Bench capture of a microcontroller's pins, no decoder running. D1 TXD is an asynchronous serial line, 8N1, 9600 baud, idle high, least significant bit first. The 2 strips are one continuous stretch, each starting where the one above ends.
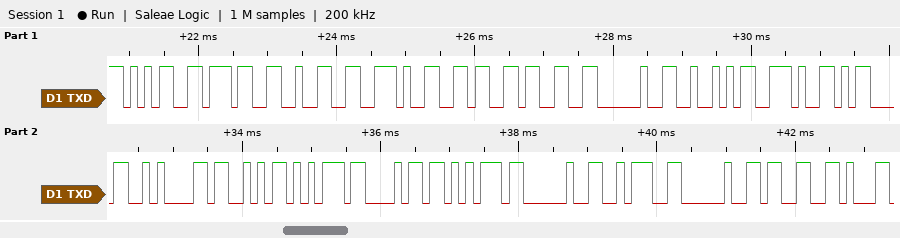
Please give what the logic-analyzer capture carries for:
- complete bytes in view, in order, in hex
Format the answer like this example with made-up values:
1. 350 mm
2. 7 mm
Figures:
1. 35 37 32 2E 36 33 20 52 2E 0D 0A 53 75 68 75 20 3A 20 33
